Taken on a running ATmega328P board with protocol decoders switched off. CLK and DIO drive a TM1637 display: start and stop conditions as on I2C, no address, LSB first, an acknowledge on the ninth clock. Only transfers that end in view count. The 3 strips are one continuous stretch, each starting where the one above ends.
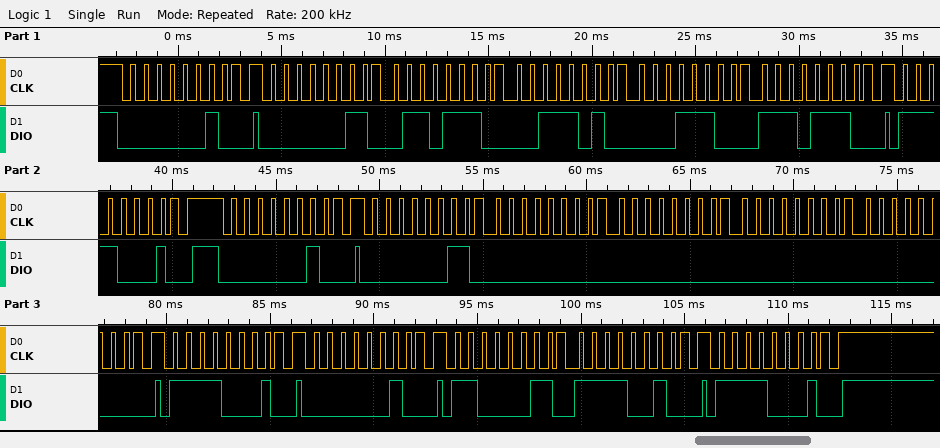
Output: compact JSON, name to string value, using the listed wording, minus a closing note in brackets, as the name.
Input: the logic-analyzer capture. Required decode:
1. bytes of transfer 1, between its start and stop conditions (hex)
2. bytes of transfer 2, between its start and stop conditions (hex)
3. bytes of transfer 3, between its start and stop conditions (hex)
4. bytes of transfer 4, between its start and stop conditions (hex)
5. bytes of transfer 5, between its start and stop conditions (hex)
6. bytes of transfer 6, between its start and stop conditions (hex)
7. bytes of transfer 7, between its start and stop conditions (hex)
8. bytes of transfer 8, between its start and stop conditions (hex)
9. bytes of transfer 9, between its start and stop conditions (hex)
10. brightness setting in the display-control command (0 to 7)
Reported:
{"bytes of transfer 1, between its start and stop conditions": "40", "bytes of transfer 2, between its start and stop conditions": "C0 76 5C 38 77", "bytes of transfer 3, between its start and stop conditions": "8F", "bytes of transfer 4, between its start and stop conditions": "40", "bytes of transfer 5, between its start and stop conditions": "C0 00 00 00 00", "bytes of transfer 6, between its start and stop conditions": "8F", "bytes of transfer 7, between its start and stop conditions": "40", "bytes of transfer 8, between its start and stop conditions": "C3 4F", "bytes of transfer 9, between its start and stop conditions": "8F", "brightness setting in the display-control command": "7"}
